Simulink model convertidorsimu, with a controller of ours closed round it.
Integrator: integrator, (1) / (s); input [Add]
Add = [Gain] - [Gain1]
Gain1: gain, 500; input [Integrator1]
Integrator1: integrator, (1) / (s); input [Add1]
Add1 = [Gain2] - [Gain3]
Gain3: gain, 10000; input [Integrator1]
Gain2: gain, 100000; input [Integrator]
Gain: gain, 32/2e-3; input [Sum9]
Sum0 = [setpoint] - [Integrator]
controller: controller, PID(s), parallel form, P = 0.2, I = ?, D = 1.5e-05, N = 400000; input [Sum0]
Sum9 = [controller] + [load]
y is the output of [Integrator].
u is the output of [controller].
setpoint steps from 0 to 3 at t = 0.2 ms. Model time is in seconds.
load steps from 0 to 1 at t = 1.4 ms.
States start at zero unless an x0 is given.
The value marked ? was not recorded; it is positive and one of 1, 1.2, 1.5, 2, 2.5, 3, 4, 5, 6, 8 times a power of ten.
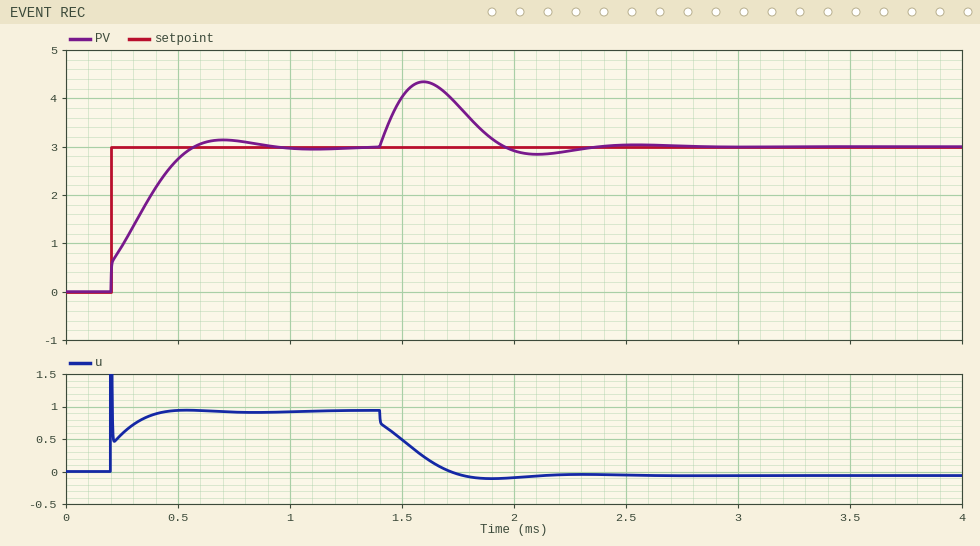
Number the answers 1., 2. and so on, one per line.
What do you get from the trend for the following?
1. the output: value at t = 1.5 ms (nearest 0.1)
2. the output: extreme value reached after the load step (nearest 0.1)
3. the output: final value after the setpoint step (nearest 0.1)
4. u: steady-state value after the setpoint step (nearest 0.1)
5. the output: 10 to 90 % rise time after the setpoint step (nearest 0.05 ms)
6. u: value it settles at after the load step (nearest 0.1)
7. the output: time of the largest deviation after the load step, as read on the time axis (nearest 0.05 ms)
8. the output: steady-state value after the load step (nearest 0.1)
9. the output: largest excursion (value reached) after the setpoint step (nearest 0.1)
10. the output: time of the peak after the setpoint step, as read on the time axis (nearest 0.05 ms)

1. 4.0
2. 4.3
3. 3.0
4. 0.9
5. 0.30 ms
6. -0.1
7. 1.60 ms
8. 3.0
9. 3.1
10. 0.70 ms
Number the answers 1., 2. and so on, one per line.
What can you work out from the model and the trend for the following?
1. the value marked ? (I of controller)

1. 2500
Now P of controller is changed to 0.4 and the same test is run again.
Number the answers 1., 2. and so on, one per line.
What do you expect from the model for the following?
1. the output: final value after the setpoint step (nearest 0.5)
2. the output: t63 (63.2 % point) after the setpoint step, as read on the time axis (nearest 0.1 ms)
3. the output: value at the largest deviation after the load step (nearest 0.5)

1. 3.0
2. 0.3 ms
3. 4.0
